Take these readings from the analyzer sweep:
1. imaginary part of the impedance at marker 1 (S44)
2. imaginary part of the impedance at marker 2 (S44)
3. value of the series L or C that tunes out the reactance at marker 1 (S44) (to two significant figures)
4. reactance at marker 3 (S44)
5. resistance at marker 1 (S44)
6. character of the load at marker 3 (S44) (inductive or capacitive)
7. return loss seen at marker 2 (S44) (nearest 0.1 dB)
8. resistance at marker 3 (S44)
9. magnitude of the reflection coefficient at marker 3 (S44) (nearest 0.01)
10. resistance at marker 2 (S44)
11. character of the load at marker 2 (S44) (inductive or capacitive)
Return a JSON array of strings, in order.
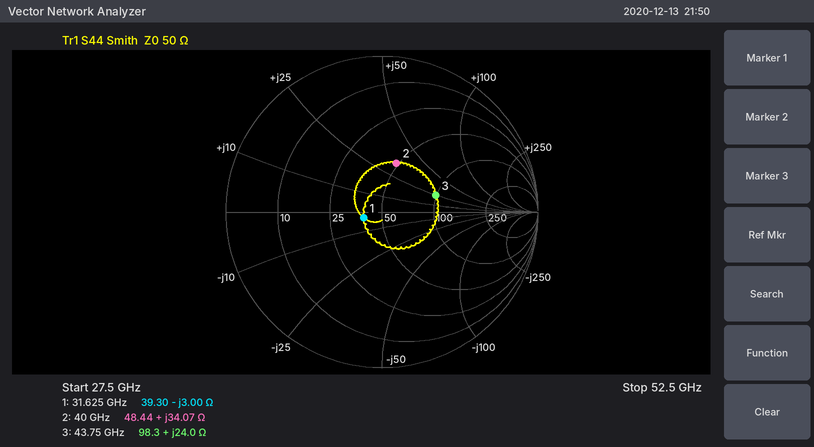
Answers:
["-3.00 Ω", "+34.07 Ω", "15 pH", "+24.0 Ω", "39.30 Ω", "inductive", "9.7 dB", "98.3 Ω", "0.36", "48.44 Ω", "inductive"]
